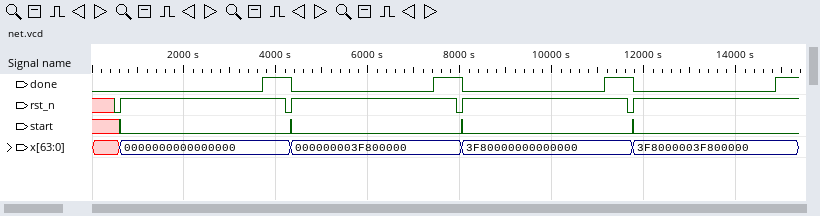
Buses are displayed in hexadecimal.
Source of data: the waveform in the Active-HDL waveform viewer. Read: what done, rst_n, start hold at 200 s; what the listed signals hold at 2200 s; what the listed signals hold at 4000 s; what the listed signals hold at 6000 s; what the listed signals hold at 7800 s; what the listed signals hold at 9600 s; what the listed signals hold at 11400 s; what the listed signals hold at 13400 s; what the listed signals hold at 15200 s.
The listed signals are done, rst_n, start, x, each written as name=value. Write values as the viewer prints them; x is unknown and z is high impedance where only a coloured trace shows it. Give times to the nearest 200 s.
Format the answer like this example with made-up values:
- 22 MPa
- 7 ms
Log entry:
- done=0, rst_n=x, start=x
- done=0, rst_n=1, start=0, x=0000000000000000
- done=1, rst_n=1, start=0, x=0000000000000000
- done=0, rst_n=1, start=0, x=000000003F800000
- done=1, rst_n=1, start=0, x=000000003F800000
- done=0, rst_n=1, start=0, x=3F80000000000000
- done=1, rst_n=1, start=0, x=3F80000000000000
- done=0, rst_n=1, start=0, x=3F8000003F800000
- done=1, rst_n=1, start=0, x=3F8000003F800000
